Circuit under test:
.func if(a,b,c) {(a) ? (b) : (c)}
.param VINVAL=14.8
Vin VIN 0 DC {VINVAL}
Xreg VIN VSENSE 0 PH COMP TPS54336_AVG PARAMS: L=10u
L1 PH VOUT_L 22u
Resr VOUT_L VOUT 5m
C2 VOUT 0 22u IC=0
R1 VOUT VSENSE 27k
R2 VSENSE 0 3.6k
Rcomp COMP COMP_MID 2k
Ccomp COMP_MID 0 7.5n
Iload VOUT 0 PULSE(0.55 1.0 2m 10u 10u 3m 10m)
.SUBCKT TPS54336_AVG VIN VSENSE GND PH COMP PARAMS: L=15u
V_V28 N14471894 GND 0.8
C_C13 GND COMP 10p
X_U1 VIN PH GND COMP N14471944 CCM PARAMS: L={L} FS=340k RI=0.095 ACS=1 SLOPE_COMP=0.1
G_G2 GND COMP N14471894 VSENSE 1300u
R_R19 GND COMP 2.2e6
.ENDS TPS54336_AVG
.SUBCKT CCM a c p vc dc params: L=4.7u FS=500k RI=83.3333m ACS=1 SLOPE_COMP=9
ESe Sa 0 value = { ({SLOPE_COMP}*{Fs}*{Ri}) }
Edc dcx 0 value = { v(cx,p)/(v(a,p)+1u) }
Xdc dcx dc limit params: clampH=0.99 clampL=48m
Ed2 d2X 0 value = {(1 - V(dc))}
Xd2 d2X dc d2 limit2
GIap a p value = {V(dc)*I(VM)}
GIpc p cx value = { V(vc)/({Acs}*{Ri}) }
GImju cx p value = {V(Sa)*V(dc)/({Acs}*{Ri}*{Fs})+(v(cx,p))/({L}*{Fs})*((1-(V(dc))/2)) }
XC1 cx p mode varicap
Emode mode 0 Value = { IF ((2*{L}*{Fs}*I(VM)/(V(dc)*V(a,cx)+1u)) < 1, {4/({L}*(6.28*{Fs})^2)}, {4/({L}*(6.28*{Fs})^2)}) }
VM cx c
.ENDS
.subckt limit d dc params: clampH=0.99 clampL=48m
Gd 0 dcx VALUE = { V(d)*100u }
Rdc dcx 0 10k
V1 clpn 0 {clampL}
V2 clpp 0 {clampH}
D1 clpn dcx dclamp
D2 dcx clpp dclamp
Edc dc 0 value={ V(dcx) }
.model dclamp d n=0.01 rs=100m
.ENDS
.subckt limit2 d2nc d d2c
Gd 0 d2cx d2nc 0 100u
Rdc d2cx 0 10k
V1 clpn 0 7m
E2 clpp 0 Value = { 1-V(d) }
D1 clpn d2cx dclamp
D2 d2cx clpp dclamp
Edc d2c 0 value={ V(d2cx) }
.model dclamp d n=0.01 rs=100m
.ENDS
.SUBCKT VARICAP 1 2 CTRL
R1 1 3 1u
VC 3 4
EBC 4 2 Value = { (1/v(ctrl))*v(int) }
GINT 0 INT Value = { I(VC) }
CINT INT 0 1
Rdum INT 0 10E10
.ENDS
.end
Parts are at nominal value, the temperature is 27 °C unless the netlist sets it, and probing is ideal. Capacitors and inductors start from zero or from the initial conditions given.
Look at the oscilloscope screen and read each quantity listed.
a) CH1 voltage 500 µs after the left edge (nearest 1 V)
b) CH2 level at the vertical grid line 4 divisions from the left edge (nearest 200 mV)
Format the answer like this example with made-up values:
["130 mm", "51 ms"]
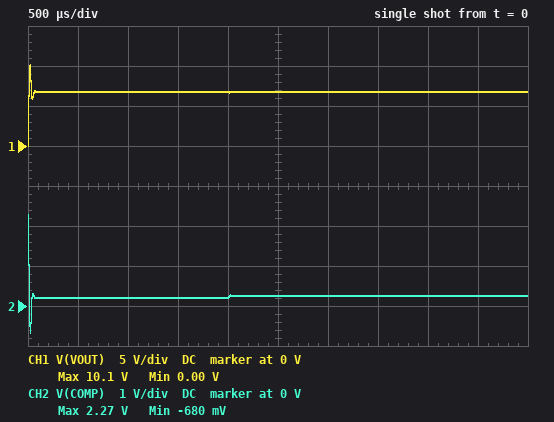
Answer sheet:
["7 V", "200 mV"]
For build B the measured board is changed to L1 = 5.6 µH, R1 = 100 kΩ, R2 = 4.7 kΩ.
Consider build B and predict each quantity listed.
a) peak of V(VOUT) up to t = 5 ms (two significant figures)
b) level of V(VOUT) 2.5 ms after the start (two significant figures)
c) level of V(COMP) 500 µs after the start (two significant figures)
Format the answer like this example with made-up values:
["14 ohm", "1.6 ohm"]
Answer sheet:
["23 V", "18 V", "310 mV"]
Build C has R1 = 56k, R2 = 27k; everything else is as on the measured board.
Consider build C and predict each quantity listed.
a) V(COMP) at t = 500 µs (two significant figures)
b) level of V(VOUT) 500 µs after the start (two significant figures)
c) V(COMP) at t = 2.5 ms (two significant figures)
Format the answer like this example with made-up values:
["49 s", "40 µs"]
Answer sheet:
["120 mV", "2.5 V", "160 mV"]
